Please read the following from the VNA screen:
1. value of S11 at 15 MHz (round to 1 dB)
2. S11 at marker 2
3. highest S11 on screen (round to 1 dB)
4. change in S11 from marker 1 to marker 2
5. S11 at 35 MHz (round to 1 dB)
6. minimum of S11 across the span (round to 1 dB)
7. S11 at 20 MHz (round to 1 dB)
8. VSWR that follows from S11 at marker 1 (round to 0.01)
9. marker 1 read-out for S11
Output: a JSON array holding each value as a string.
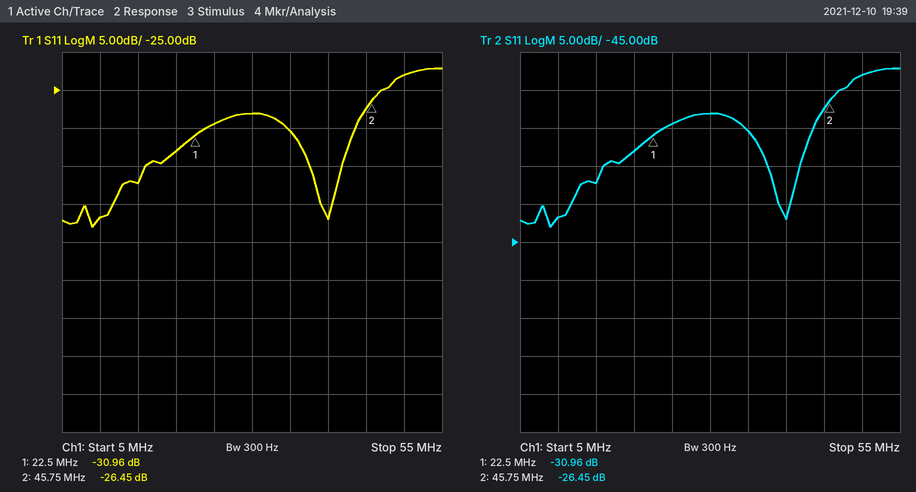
["-37 dB", "-26.45 dB", "-22 dB", "4.51 dB", "-30 dB", "-43 dB", "-33 dB", "1.06", "-30.96 dB"]
